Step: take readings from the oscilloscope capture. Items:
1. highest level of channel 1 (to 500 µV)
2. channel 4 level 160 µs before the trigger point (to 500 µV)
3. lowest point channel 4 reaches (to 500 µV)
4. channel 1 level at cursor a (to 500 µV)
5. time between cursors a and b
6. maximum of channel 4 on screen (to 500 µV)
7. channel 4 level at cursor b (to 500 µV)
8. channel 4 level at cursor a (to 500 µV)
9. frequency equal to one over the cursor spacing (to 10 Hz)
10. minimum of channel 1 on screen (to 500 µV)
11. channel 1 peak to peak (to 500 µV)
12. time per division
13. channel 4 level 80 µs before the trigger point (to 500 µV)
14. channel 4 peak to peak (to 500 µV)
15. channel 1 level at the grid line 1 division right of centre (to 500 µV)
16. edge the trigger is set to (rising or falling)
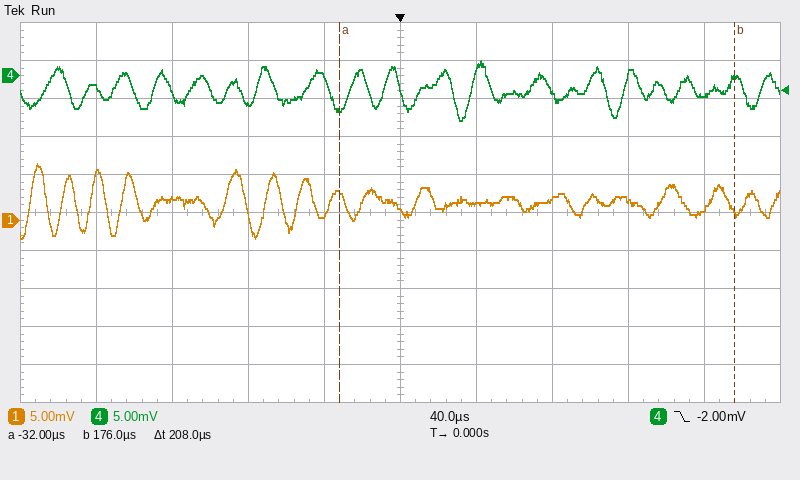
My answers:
7.5 mV
-1.5 mV
-6.0 mV
3.5 mV
208 µs
2.0 mV
-500 µV
-4.5 mV
4.81 kHz
-2.5 mV
10.0 mV
40 µs
-3.5 mV
8.0 mV
2.0 mV
falling
